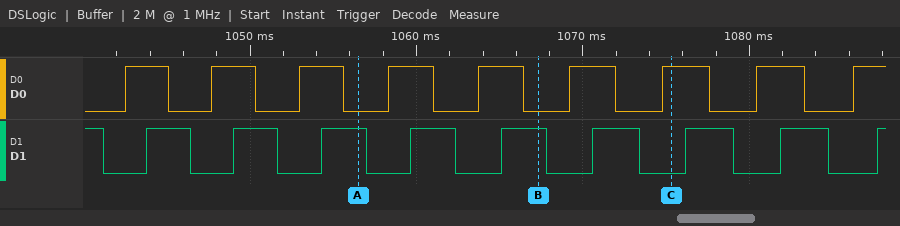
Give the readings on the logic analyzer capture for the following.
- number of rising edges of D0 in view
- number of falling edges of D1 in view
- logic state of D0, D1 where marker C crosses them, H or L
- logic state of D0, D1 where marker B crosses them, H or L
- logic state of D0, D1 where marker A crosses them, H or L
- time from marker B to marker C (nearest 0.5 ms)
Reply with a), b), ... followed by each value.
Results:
a) 9
b) 9
c) D0=H, D1=L
d) D0=L, D1=H
e) D0=L, D1=H
f) 8 ms
